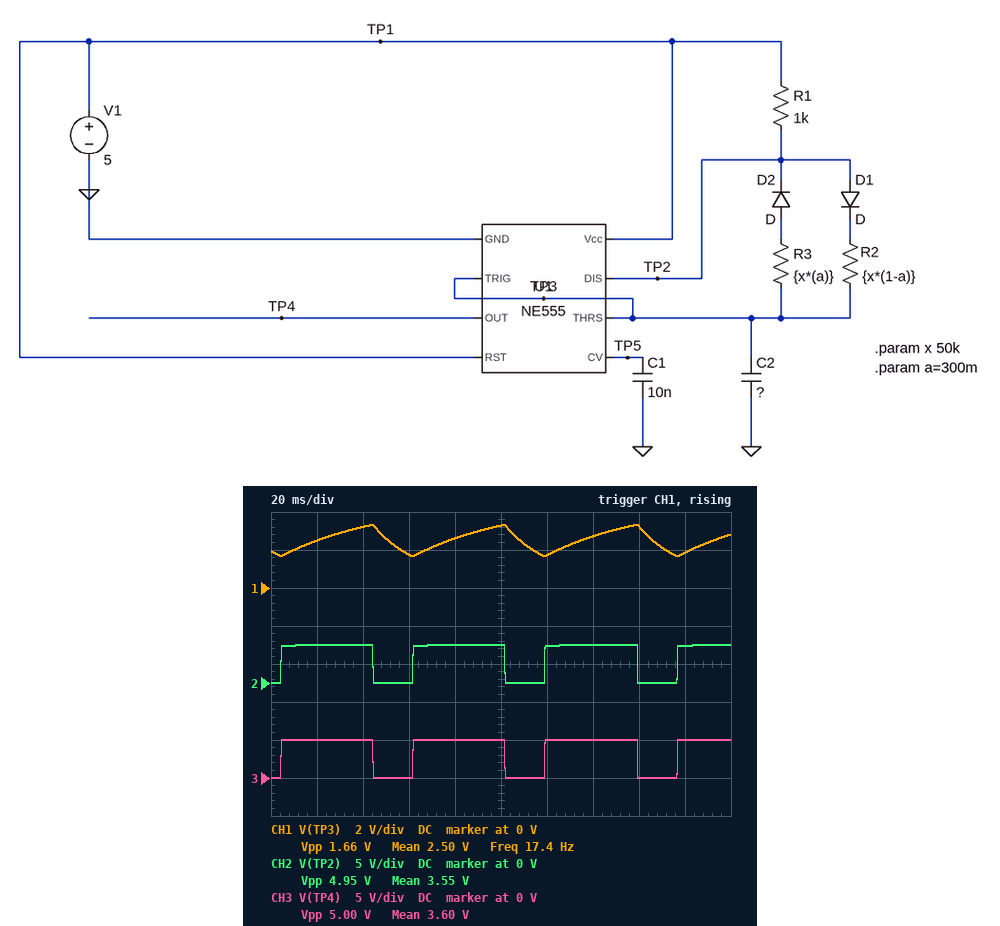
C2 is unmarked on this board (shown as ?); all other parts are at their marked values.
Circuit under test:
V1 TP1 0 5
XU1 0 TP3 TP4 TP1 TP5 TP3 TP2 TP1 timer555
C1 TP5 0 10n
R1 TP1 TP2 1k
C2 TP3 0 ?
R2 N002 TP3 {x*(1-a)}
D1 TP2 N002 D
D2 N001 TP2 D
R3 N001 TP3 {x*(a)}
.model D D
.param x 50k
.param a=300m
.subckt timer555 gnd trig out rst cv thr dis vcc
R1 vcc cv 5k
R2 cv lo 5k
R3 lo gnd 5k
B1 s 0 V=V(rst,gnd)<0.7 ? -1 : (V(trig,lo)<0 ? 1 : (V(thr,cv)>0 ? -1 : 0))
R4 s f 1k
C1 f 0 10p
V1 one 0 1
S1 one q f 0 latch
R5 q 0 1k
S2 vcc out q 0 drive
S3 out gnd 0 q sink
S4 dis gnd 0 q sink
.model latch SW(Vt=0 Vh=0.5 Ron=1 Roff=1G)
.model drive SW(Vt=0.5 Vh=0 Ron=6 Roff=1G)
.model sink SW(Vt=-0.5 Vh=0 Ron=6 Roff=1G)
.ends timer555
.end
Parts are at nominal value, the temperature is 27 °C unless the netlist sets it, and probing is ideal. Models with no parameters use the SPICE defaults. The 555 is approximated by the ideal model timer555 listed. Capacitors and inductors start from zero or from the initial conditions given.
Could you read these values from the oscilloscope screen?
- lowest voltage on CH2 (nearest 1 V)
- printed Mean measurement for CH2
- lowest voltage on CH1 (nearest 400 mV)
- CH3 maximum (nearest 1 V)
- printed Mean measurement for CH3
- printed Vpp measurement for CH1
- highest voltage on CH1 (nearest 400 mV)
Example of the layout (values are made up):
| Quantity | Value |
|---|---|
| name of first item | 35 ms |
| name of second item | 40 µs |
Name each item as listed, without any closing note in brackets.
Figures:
| Quantity | Value |
|---|---|
| lowest voltage on CH2 | 0 V |
| printed Mean measurement for CH2 | 3.55 V |
| lowest voltage on CH1 | 1.6 V |
| CH3 maximum | 5 V |
| printed Mean measurement for CH3 | 3.60 V |
| printed Vpp measurement for CH1 | 1.66 V |
| highest voltage on CH1 | 3.2 V |
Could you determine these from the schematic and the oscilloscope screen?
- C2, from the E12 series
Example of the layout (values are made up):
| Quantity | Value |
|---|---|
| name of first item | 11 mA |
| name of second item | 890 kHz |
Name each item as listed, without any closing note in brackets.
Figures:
| Quantity | Value |
|---|---|
| C2, from the E12 series | 1.2 µF |
